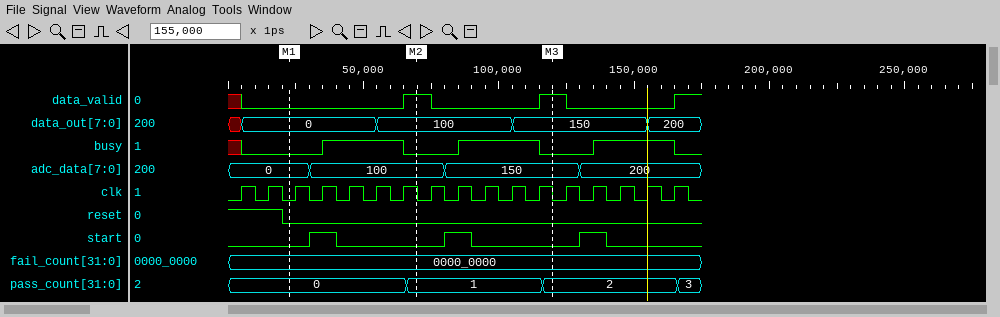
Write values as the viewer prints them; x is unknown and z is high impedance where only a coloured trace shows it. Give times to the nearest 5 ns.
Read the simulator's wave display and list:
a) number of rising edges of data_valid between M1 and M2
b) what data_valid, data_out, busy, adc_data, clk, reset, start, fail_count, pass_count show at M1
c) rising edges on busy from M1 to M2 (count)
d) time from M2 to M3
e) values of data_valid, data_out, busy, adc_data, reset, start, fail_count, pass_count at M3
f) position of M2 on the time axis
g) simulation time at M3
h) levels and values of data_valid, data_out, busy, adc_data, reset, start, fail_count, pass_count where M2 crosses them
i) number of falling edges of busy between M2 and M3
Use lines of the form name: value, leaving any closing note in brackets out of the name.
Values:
number of rising edges of data_valid between M1 and M2: 1
what data_valid, data_out, busy, adc_data, clk, reset, start, fail_count, pass_count show at M1: data_valid=0, data_out=0, busy=0, adc_data=0, clk=0, reset=0, start=0, fail_count=0000_0000, pass_count=0
rising edges on busy from M1 to M2: 1
time from M2 to M3: 50 ns
values of data_valid, data_out, busy, adc_data, reset, start, fail_count, pass_count at M3: data_valid=1, data_out=150, busy=0, adc_data=150, reset=0, start=0, fail_count=0000_0000, pass_count=2
position of M2 on the time axis: 70 ns
simulation time at M3: 120 ns
levels and values of data_valid, data_out, busy, adc_data, reset, start, fail_count, pass_count where M2 crosses them: data_valid=1, data_out=100, busy=0, adc_data=100, reset=0, start=0, fail_count=0000_0000, pass_count=1
number of falling edges of busy between M2 and M3: 1
